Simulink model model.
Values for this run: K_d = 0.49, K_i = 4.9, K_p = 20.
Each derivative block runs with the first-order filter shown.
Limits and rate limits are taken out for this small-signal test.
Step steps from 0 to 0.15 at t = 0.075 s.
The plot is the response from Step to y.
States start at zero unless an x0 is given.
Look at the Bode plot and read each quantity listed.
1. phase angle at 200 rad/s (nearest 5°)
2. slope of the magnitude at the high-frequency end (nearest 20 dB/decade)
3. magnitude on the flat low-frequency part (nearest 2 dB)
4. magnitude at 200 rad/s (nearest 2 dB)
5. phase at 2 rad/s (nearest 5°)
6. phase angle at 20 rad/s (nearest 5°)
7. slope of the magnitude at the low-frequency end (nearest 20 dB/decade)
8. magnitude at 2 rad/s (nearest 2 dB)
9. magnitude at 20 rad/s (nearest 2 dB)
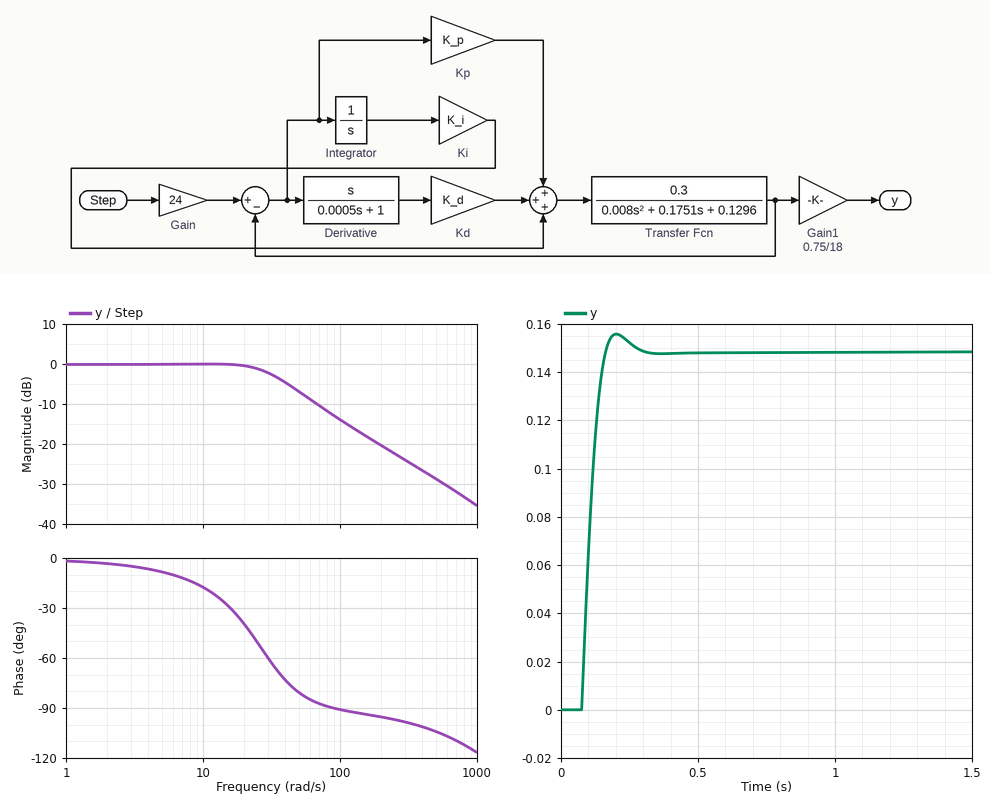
-95°
-20 dB/decade
0 dB
-20 dB
-5°
-40°
0 dB/decade
0 dB
0 dB
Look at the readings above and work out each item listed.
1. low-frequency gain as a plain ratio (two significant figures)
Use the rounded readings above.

1.0
